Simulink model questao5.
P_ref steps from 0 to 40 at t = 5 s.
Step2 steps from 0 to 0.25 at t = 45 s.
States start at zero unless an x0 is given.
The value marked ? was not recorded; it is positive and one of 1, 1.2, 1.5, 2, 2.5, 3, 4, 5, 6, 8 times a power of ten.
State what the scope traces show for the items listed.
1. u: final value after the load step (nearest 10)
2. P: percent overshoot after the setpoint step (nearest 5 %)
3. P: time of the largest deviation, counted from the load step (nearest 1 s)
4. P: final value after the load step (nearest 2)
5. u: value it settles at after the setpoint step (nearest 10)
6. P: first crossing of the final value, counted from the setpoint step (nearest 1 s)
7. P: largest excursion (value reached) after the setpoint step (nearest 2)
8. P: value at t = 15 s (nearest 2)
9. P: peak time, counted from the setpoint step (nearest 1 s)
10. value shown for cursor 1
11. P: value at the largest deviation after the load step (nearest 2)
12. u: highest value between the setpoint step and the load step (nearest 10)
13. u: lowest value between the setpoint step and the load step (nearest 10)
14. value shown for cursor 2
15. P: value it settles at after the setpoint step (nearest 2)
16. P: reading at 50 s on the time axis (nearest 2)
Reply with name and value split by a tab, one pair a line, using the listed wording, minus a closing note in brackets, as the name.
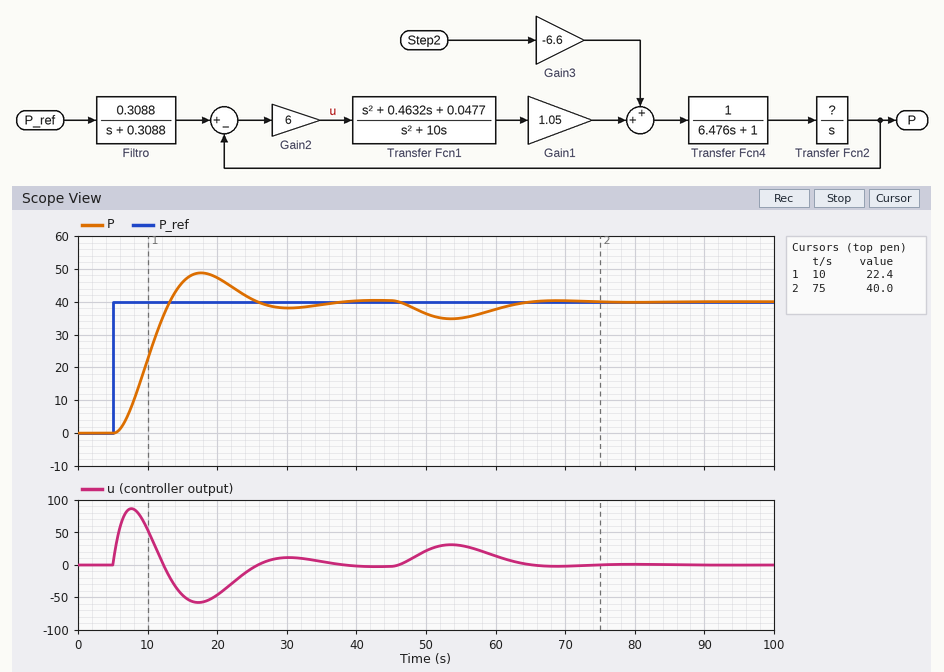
u: final value after the load step	0
P: percent overshoot after the setpoint step	20 %
P: time of the largest deviation, counted from the load step	9 s
P: final value after the load step	40
u: value it settles at after the setpoint step	0
P: first crossing of the final value, counted from the setpoint step	8 s
P: largest excursion (value reached) after the setpoint step	48
P: value at t = 15 s	46
P: peak time, counted from the setpoint step	13 s
value shown for cursor 1	22.4
P: value at the largest deviation after the load step	34
u: highest value between the setpoint step and the load step	90
u: lowest value between the setpoint step and the load step	-60
value shown for cursor 2	40.0
P: value it settles at after the setpoint step	40
P: reading at 50 s on the time axis	36
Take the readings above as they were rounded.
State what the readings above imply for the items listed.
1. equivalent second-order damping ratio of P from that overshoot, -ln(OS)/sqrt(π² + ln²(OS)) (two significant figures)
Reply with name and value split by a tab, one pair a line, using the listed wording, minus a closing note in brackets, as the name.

equivalent second-order damping ratio of P from that overshoot, -ln(OS)/sqrt(π² + ln²(OS))	0.46
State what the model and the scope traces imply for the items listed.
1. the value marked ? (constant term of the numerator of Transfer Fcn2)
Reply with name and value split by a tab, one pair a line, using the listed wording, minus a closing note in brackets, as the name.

the value marked ?	2.5
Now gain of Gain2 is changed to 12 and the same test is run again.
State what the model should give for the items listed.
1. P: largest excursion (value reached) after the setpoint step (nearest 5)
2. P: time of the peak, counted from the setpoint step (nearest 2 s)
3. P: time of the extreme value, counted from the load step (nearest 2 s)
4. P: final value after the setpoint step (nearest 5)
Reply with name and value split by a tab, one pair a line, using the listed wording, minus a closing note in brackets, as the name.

P: largest excursion (value reached) after the setpoint step	45
P: time of the peak, counted from the setpoint step	10 s
P: time of the extreme value, counted from the load step	6 s
P: final value after the setpoint step	40
